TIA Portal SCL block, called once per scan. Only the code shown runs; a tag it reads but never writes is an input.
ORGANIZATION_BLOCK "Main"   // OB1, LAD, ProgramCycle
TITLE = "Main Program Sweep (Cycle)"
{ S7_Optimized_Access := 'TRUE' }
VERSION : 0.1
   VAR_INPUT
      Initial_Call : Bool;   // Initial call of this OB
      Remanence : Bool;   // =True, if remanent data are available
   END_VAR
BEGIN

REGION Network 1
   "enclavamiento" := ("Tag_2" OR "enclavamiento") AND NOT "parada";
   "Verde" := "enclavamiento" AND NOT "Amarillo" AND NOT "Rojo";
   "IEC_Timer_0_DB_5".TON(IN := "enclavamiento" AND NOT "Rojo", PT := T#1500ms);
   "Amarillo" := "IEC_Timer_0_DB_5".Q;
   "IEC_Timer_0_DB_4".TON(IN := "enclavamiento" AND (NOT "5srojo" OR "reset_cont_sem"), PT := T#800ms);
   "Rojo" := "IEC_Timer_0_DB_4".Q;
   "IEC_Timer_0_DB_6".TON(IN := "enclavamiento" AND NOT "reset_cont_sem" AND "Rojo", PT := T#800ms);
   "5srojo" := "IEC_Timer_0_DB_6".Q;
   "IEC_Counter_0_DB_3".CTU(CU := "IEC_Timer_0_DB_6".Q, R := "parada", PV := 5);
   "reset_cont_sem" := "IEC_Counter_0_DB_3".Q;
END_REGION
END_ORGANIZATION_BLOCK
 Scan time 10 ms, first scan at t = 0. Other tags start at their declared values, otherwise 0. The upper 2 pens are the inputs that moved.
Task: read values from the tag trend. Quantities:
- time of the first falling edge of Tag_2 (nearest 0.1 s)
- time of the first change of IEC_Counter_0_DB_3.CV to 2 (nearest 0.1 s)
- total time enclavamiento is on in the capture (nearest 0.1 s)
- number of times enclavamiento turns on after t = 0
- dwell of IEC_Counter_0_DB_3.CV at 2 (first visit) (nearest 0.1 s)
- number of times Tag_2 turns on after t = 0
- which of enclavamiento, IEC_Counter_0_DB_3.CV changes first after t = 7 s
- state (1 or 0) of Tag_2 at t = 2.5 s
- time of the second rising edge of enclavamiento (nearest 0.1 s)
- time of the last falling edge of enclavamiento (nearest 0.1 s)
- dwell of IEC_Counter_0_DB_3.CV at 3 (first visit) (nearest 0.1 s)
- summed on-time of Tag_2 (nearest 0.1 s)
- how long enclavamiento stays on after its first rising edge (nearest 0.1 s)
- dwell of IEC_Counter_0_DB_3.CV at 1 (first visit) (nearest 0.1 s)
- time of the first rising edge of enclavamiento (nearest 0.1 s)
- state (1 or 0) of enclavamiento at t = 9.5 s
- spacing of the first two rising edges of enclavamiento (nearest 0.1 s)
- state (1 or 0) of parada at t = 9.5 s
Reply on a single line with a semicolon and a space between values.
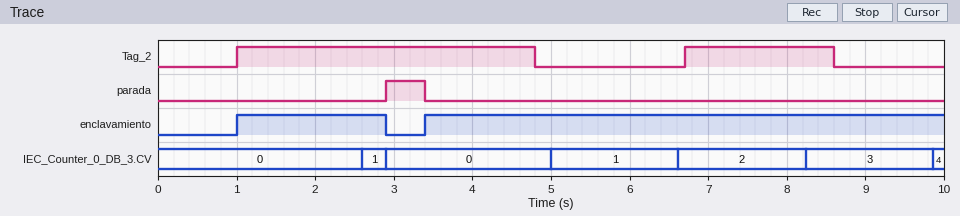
4.8 s; 6.6 s; 8.5 s; 2; 1.6 s; 2; IEC_Counter_0_DB_3.CV; 1; 3.4 s; 2.9 s; 1.6 s; 5.7 s; 1.9 s; 0.3 s; 1.0 s; 1; 2.4 s; 0
